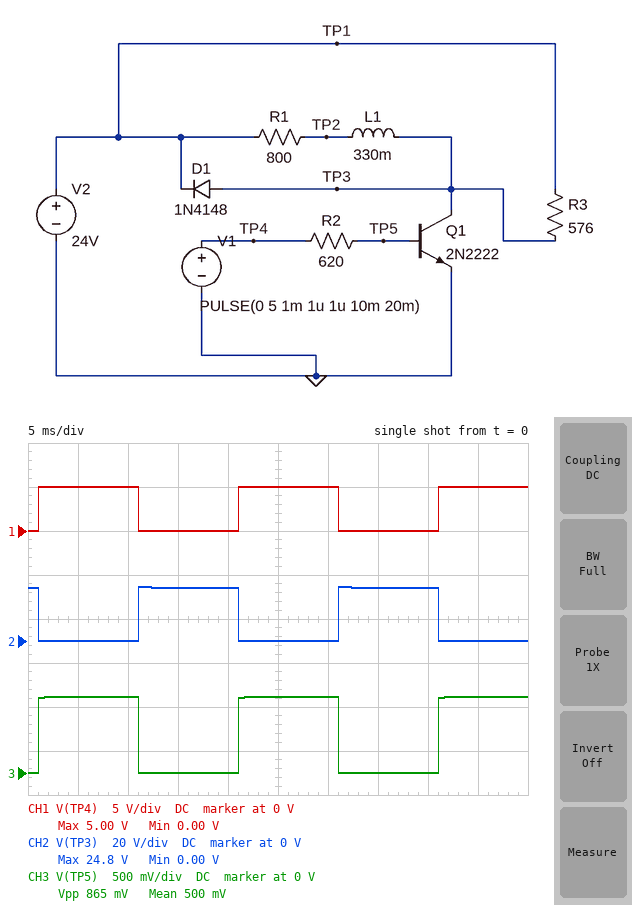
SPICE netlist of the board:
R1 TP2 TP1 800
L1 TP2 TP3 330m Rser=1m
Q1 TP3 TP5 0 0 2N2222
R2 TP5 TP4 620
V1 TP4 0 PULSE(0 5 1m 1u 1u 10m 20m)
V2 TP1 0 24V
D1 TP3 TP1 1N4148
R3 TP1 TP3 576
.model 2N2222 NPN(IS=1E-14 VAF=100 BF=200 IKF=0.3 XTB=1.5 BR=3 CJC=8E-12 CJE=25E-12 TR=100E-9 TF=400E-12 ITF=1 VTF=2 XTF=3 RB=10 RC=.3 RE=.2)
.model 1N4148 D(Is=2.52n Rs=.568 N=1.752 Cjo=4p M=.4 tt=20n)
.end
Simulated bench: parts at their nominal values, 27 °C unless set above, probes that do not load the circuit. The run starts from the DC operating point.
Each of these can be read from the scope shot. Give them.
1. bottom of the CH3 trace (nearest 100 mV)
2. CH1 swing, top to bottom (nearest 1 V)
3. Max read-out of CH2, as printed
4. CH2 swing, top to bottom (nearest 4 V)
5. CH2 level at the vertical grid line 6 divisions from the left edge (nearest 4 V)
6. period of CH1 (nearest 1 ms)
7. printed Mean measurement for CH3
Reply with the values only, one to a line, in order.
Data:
0 V
5 V
24.8 V
24 V
0 V
20 ms
500 mV
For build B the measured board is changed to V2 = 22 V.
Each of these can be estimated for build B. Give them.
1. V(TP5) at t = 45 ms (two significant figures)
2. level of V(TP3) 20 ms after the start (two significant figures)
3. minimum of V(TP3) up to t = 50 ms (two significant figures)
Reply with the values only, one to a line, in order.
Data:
860 mV
22 V
55 mV
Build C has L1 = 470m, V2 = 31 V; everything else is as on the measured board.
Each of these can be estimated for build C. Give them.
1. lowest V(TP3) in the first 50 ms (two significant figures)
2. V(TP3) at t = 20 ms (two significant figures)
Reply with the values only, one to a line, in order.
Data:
70 mV
31 V
